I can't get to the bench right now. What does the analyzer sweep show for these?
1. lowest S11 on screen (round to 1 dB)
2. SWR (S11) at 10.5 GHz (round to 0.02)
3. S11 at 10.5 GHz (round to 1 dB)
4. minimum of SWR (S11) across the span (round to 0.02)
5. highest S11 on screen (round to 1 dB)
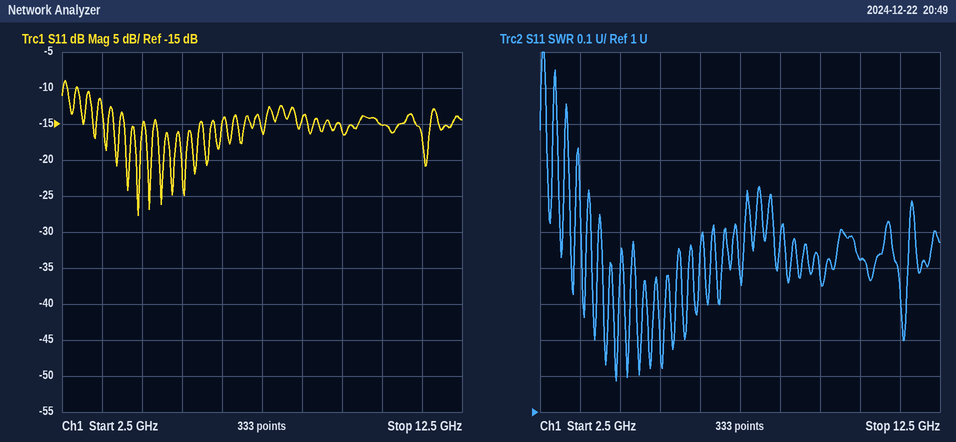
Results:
-28 dB
1.42
-15 dB
1.08
-9 dB
